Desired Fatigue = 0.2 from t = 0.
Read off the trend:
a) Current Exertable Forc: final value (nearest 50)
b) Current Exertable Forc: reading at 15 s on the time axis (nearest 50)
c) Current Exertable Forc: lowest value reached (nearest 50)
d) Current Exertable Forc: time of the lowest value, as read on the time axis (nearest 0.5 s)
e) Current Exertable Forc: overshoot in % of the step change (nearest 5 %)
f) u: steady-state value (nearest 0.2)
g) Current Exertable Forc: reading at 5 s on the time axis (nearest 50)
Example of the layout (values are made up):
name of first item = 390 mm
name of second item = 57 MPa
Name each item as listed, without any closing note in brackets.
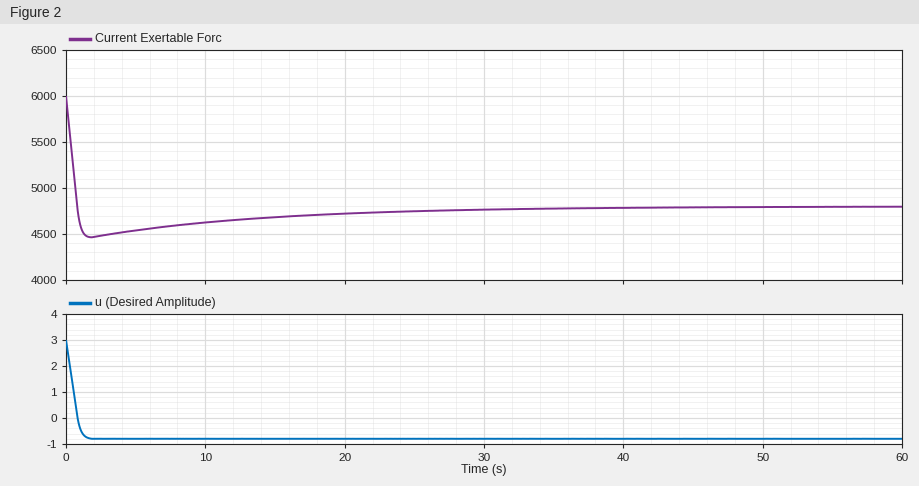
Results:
Current Exertable Forc: final value = 4800
Current Exertable Forc: reading at 15 s on the time axis = 4700
Current Exertable Forc: lowest value reached = 4450
Current Exertable Forc: time of the lowest value, as read on the time axis = 2.0 s
Current Exertable Forc: overshoot in % of the step change = 30 %
u: steady-state value = -0.8
Current Exertable Forc: reading at 5 s on the time axis = 4550
